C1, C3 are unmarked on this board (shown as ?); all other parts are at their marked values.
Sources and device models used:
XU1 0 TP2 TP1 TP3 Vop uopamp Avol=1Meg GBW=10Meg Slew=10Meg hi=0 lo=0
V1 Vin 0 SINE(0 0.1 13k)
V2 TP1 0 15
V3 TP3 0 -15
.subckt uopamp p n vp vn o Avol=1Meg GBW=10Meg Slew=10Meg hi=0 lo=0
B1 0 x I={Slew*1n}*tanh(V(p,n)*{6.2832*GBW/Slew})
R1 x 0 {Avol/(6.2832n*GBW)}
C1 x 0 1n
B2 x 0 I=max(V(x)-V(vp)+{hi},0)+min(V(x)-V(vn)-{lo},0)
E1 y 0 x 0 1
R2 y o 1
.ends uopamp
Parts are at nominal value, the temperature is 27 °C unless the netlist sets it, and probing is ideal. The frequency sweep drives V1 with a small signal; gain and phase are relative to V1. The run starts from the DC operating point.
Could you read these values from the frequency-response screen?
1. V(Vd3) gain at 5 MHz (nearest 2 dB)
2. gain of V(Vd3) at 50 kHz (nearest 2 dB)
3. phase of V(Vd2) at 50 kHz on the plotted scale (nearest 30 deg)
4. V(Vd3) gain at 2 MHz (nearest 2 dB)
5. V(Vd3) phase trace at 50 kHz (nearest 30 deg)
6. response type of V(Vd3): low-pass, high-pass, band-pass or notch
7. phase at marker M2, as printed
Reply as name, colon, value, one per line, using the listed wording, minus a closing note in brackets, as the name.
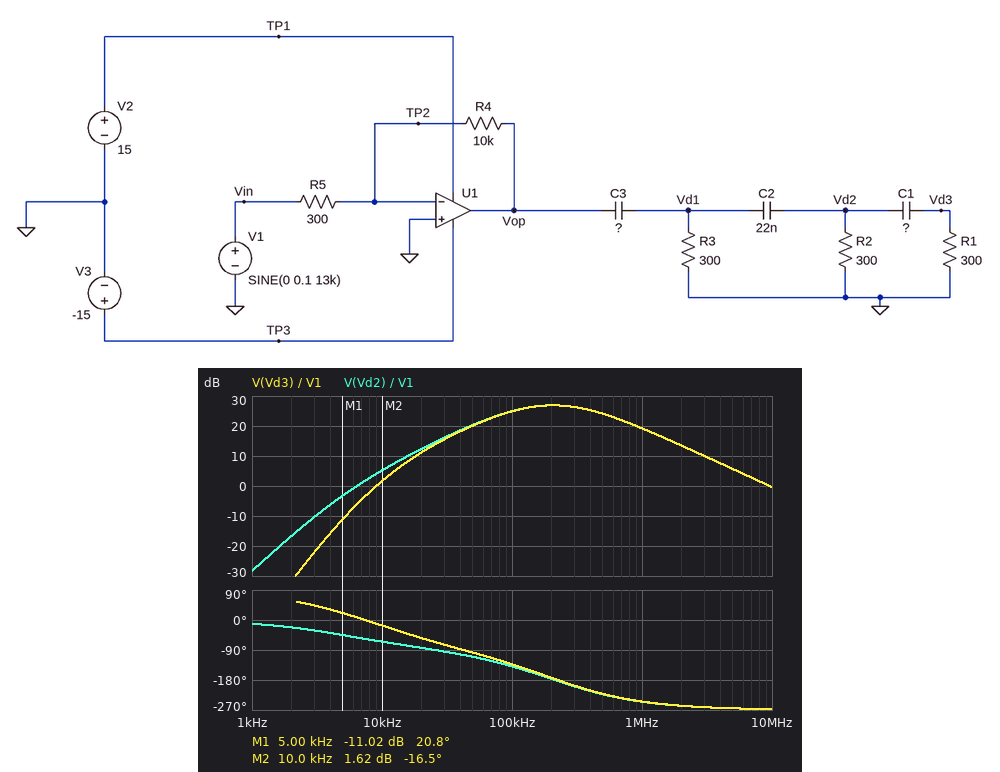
V(Vd3) gain at 5 MHz: 6 dB
gain of V(Vd3) at 50 kHz: 20 dB
phase of V(Vd2) at 50 kHz on the plotted scale: -120 deg
V(Vd3) gain at 2 MHz: 14 dB
V(Vd3) phase trace at 50 kHz: -90 deg
response type of V(Vd3): low-pass, high-pass, band-pass or notch: band-pass
phase at marker M2, as printed: -16.5 deg
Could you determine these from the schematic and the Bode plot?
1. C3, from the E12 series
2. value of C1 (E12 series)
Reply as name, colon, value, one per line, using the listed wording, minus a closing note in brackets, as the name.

C3, from the E12 series: 15 nF
value of C1: 47 nF
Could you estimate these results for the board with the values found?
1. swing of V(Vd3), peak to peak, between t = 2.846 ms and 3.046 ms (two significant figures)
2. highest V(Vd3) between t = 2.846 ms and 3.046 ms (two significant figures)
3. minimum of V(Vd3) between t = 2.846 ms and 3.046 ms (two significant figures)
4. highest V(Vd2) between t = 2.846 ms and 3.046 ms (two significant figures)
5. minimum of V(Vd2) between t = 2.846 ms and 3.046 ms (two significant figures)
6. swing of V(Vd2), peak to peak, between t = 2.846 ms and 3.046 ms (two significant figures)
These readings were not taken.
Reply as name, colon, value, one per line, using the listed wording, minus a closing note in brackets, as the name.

swing of V(Vd3), peak to peak, between t = 2.846 ms and 3.046 ms: 380 mV
highest V(Vd3) between t = 2.846 ms and 3.046 ms: 190 mV
minimum of V(Vd3) between t = 2.846 ms and 3.046 ms: -190 mV
highest V(Vd2) between t = 2.846 ms and 3.046 ms: 250 mV
minimum of V(Vd2) between t = 2.846 ms and 3.046 ms: -250 mV
swing of V(Vd2), peak to peak, between t = 2.846 ms and 3.046 ms: 500 mV
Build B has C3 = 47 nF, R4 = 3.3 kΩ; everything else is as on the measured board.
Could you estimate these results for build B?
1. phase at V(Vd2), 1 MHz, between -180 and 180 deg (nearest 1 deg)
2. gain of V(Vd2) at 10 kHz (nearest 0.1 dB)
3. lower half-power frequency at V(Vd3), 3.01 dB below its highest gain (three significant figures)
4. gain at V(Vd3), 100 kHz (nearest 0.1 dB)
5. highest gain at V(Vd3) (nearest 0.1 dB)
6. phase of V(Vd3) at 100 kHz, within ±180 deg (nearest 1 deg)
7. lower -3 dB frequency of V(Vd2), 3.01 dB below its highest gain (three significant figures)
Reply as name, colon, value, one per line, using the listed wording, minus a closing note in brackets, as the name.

phase at V(Vd2), 1 MHz, between -180 and 180 deg: 134 deg
gain of V(Vd2) at 10 kHz: 3.1 dB
lower half-power frequency at V(Vd3), 3.01 dB below its highest gain: 69.3 kHz
gain at V(Vd3), 100 kHz: 18.6 dB
highest gain at V(Vd3): 20.0 dB
phase of V(Vd3) at 100 kHz, within ±180 deg: -141 deg
lower -3 dB frequency of V(Vd2), 3.01 dB below its highest gain: 67.8 kHz
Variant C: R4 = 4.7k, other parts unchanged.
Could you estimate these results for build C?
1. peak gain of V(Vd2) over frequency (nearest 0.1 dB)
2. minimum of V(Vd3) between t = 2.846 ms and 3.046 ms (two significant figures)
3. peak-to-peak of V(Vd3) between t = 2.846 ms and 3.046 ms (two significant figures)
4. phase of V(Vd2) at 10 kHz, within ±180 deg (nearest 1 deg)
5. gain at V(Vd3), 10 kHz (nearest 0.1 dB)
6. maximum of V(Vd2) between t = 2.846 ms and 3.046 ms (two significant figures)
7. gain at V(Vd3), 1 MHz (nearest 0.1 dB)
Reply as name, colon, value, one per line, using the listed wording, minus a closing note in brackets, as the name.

peak gain of V(Vd2) over frequency: 22.0 dB
minimum of V(Vd3) between t = 2.846 ms and 3.046 ms: -89 mV
peak-to-peak of V(Vd3) between t = 2.846 ms and 3.046 ms: 180 mV
phase of V(Vd2) at 10 kHz, within ±180 deg: -64 deg
gain at V(Vd3), 10 kHz: -4.9 dB
maximum of V(Vd2) between t = 2.846 ms and 3.046 ms: 120 mV
gain at V(Vd3), 1 MHz: 18.0 dB
